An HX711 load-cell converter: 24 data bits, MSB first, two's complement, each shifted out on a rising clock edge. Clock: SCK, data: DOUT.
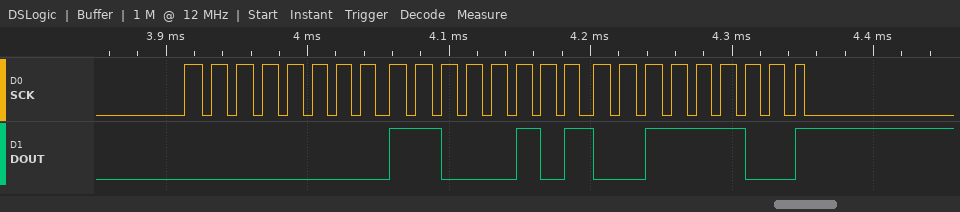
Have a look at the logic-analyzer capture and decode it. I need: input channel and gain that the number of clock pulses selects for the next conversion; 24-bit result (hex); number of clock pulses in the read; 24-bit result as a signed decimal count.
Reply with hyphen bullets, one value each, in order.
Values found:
- channel A, gain 128
- 0x00C53C
- 25
- 50492
